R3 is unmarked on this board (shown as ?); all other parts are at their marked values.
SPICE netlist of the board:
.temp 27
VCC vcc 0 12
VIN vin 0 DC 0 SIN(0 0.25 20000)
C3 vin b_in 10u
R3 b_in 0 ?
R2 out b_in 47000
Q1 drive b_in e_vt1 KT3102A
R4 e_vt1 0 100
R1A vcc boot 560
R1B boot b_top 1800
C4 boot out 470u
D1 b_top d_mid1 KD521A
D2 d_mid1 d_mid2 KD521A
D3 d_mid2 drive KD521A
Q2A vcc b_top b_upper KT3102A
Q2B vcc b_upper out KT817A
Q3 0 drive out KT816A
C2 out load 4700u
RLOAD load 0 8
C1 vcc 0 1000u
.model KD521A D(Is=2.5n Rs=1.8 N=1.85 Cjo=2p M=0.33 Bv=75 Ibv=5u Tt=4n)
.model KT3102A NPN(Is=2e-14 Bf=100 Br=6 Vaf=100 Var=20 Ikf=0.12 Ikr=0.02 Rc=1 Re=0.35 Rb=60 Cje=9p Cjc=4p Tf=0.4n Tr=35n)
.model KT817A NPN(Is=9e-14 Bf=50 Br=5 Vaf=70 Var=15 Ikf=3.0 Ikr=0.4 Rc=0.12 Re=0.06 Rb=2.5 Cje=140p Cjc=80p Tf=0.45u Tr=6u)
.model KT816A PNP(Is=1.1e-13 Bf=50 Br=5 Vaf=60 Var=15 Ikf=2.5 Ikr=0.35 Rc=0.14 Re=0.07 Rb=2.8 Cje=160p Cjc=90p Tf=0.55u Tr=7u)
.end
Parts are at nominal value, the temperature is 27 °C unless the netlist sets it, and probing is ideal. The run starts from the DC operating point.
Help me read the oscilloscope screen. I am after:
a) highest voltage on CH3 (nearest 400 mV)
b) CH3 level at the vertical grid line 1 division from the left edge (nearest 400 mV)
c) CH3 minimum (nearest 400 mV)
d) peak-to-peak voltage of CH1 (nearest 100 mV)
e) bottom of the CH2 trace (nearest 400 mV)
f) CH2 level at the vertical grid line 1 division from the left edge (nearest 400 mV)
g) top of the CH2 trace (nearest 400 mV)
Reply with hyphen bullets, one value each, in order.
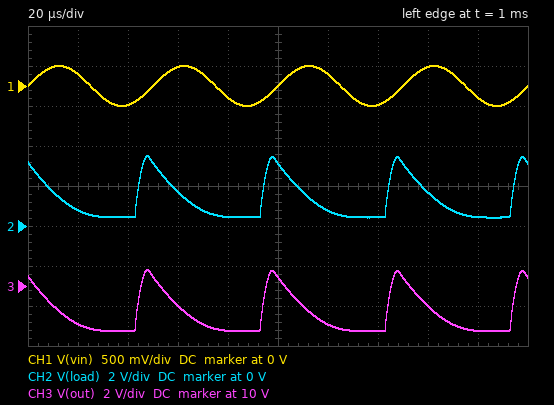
- 10.8 V
- 8.0 V
- 7.6 V
- 500 mV
- 400 mV
- 800 mV
- 3.6 V
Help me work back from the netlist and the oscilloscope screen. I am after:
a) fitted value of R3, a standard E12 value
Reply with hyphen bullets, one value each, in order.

- 6.8 kΩ
